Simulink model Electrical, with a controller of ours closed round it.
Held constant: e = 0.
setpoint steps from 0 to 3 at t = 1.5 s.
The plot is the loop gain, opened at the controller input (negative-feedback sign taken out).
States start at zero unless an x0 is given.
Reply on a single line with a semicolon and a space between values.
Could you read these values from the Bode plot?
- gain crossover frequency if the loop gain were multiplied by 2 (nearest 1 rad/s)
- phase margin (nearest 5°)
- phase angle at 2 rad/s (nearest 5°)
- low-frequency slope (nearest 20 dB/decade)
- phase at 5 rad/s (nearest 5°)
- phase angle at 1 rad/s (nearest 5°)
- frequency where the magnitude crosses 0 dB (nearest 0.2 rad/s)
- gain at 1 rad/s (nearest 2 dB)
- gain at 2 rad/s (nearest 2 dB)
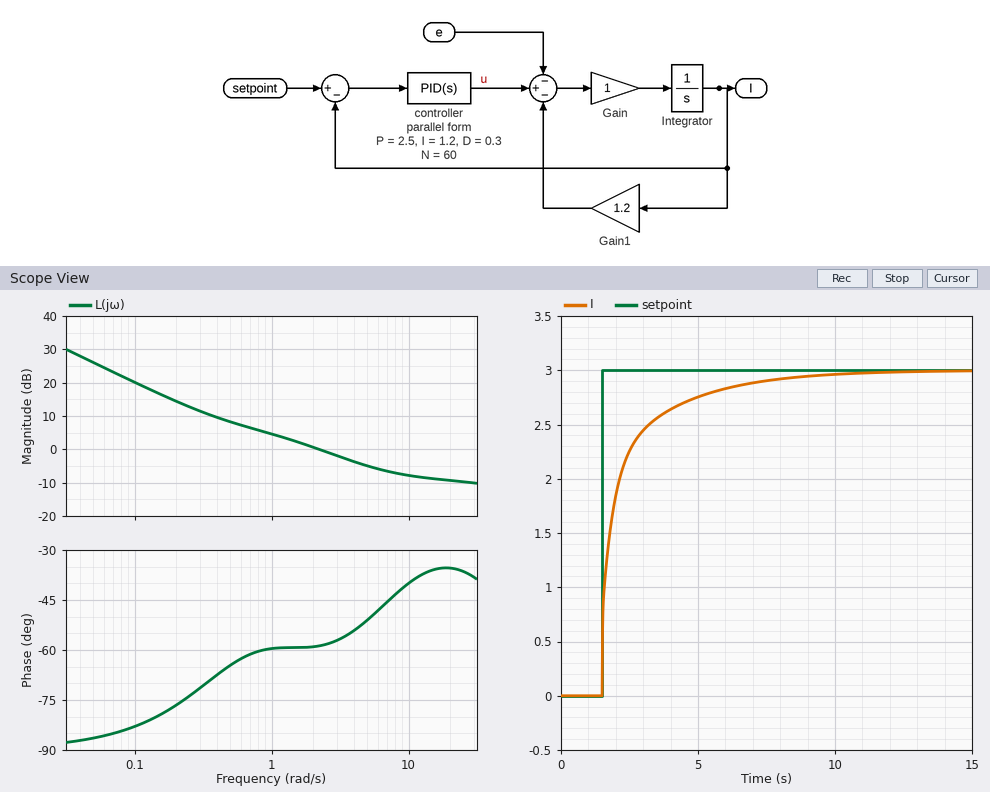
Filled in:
6 rad/s; 120°; -60°; -20 dB/decade; -50°; -60°; 2.2 rad/s; 4 dB; 0 dB
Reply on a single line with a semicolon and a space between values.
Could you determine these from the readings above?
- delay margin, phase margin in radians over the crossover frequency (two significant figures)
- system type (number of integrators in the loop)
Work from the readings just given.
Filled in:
0.95 s; 1
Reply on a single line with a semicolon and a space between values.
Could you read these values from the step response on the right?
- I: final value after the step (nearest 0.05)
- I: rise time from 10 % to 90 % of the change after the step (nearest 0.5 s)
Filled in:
3.00; 3.0 s
